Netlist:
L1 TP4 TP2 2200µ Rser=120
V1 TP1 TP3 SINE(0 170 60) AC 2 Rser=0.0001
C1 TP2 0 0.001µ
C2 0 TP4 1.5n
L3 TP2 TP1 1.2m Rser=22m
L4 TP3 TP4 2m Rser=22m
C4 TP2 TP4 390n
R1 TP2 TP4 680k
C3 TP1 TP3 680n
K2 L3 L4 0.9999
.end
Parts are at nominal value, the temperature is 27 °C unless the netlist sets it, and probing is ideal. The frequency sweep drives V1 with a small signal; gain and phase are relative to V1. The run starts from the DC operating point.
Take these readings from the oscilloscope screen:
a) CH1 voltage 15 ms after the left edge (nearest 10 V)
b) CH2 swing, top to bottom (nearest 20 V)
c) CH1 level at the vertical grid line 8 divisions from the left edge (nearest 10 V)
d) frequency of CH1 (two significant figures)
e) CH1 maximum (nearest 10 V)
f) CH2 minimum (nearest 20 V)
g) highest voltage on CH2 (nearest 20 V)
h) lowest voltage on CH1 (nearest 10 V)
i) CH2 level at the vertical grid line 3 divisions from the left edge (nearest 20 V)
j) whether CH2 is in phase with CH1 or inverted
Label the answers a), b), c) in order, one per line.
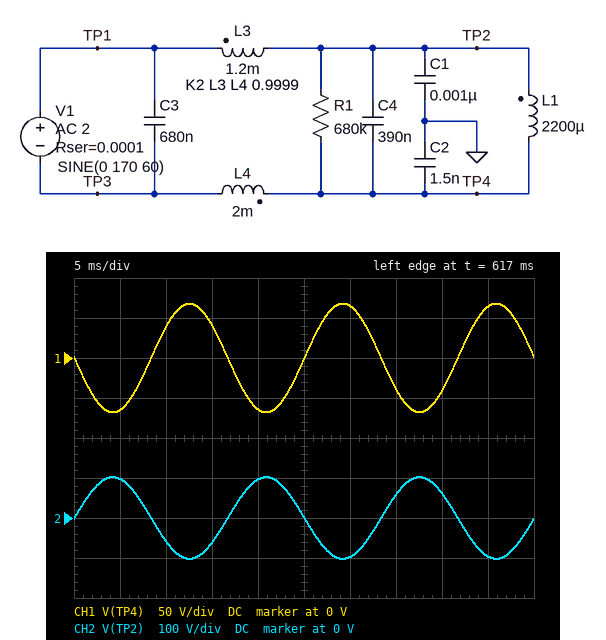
a) 40 V
b) 200 V
c) -40 V
d) 60 Hz
e) 70 V
f) -100 V
g) 100 V
h) -70 V
i) -60 V
j) inverted
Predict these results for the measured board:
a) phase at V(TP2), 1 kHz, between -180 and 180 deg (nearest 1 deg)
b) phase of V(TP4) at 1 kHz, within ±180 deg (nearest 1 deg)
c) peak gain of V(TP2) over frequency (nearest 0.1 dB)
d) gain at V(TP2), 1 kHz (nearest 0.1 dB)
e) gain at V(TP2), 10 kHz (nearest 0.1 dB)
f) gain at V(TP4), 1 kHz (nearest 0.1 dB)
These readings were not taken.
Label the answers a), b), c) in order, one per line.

a) -19 deg
b) 161 deg
c) -4.2 dB
d) -4.4 dB
e) -21.6 dB
f) -7.9 dB
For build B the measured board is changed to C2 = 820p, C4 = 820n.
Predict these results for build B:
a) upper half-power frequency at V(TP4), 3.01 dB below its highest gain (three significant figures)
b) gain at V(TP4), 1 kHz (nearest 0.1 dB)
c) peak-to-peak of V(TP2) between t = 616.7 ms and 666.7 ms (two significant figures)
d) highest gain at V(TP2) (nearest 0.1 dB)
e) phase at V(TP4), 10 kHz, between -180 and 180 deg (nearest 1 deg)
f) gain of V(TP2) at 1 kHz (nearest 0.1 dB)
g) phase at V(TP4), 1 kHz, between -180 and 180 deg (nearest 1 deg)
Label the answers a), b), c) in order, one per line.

a) 2.95 kHz
b) -4.2 dB
c) 150 V
d) -3.9 dB
e) 5 deg
f) -6.0 dB
g) 159 deg
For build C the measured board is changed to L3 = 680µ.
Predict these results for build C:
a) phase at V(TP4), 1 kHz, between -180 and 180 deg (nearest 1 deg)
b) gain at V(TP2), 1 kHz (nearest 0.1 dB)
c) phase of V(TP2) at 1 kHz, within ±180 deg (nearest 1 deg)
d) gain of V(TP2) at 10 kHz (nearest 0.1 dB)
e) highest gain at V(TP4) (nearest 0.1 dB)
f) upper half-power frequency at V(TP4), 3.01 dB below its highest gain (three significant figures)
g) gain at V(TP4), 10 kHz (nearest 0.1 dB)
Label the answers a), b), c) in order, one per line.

a) 165 deg
b) -4.3 dB
c) -15 deg
d) -19.3 dB
e) -6.8 dB
f) 5.49 kHz
g) -22.8 dB
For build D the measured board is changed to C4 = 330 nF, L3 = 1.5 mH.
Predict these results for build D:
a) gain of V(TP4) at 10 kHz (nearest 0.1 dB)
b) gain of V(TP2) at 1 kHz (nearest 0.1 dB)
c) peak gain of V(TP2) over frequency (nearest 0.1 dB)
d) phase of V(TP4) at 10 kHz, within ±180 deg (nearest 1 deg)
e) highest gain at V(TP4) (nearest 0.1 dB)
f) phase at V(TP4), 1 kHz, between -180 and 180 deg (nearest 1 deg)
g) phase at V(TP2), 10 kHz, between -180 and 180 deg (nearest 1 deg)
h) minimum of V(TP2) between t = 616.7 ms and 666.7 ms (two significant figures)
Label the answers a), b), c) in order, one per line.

a) -24.2 dB
b) -4.6 dB
c) -4.4 dB
d) 14 deg
e) -8.0 dB
f) 159 deg
g) -166 deg
h) -100 V
